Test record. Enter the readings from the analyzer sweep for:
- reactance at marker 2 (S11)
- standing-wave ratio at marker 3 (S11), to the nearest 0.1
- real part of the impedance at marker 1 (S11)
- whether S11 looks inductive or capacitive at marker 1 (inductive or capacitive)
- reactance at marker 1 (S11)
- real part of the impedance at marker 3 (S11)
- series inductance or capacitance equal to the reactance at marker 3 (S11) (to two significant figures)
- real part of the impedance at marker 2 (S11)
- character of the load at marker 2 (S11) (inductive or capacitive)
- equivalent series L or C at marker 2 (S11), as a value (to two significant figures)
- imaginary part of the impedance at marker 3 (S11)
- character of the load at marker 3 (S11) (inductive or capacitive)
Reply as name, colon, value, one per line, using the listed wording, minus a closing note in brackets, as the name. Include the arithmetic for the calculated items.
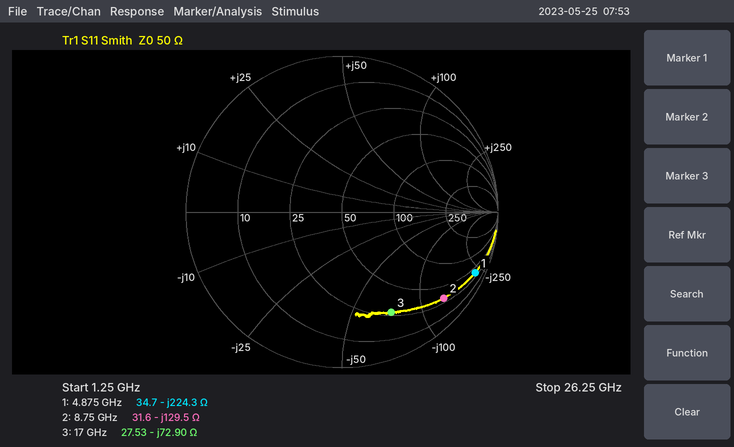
reactance at marker 2: -129.5 Ω
standing-wave ratio at marker 3 (S11), to the nearest 0.1: 6.1
real part of the impedance at marker 1: 34.7 Ω
whether S11 looks inductive or capacitive at marker 1: capacitive
reactance at marker 1: -224.3 Ω
real part of the impedance at marker 3: 27.53 Ω
series inductance or capacitance equal to the reactance at marker 3 (S11): C = 1/(2π × 17 GHz × 72.9 Ω) ≈ 128 fF, so 130 fF to two significant figures
real part of the impedance at marker 2: 31.6 Ω
character of the load at marker 2 (S11): capacitive
equivalent series L or C at marker 2 (S11), as a value: C = 1/(2π × 8.75 GHz × 129.5 Ω) ≈ 140 fF
imaginary part of the impedance at marker 3: -72.90 Ω
character of the load at marker 3 (S11): capacitive
